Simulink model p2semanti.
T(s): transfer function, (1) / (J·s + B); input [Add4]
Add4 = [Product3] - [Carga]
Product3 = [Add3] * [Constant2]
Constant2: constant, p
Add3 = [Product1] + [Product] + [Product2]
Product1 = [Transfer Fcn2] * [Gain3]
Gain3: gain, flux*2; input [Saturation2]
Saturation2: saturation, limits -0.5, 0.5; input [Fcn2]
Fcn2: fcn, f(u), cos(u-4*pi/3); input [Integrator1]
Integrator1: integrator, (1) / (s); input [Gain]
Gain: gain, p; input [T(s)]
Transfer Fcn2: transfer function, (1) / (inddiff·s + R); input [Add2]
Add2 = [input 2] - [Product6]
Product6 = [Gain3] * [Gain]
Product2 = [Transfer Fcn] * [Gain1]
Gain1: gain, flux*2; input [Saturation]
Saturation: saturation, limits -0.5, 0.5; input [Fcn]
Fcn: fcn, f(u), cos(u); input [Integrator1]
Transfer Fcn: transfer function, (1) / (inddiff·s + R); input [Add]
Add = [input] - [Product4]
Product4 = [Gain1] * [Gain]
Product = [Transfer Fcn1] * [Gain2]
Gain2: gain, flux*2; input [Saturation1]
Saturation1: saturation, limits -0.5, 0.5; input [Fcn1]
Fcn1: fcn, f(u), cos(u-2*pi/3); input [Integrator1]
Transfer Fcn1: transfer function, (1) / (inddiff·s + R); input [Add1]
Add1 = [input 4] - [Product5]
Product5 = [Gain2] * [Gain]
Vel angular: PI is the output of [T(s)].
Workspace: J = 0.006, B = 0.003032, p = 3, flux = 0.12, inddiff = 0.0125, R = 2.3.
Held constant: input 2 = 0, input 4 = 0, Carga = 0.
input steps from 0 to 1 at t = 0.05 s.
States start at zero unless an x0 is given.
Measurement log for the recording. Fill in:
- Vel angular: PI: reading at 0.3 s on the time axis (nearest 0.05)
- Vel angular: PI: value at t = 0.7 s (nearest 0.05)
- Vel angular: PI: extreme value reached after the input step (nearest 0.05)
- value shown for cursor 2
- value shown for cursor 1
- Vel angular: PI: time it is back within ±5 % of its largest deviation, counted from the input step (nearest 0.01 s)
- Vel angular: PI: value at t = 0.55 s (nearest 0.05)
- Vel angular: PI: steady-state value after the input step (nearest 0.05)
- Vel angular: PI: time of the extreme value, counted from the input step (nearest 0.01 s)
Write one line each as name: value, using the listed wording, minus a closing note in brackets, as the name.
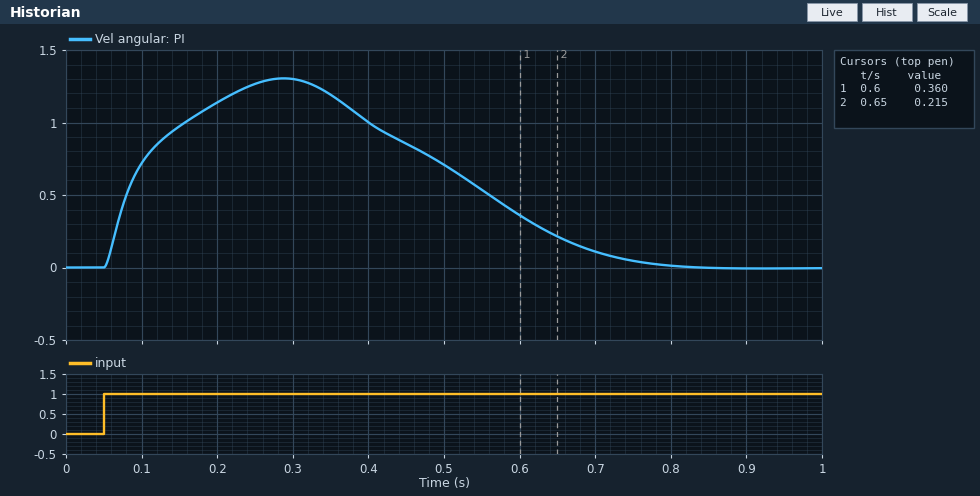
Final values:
Vel angular: PI: reading at 0.3 s on the time axis: 1.30
Vel angular: PI: value at t = 0.7 s: 0.10
Vel angular: PI: extreme value reached after the input step: 1.30
value shown for cursor 2: 0.215
value shown for cursor 1: 0.360
Vel angular: PI: time it is back within ±5 % of its largest deviation, counted from the input step: 0.68 s
Vel angular: PI: value at t = 0.55 s: 0.55
Vel angular: PI: steady-state value after the input step: 0.00
Vel angular: PI: time of the extreme value, counted from the input step: 0.24 s
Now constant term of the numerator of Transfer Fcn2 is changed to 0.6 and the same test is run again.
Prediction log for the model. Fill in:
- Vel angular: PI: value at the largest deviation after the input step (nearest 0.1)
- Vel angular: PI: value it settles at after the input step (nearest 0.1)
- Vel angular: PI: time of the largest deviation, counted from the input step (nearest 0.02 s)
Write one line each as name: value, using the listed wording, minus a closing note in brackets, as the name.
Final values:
Vel angular: PI: value at the largest deviation after the input step: 1.6
Vel angular: PI: value it settles at after the input step: 0.0
Vel angular: PI: time of the largest deviation, counted from the input step: 0.22 s
